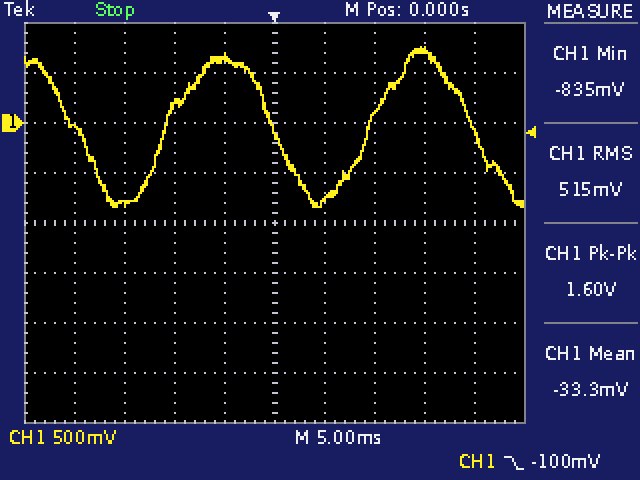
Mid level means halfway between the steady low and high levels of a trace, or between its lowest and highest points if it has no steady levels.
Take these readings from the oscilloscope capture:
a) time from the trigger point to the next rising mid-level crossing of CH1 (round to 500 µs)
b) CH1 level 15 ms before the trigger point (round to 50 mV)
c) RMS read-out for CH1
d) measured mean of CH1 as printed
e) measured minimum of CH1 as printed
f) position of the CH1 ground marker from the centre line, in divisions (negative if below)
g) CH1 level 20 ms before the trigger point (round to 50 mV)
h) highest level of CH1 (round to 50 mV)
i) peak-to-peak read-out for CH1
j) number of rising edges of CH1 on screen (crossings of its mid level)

9.5 ms
-800 mV
515 mV
-33.3 mV
-835 mV
+2.0 div
-50 mV
750 mV
1.60 V
2
